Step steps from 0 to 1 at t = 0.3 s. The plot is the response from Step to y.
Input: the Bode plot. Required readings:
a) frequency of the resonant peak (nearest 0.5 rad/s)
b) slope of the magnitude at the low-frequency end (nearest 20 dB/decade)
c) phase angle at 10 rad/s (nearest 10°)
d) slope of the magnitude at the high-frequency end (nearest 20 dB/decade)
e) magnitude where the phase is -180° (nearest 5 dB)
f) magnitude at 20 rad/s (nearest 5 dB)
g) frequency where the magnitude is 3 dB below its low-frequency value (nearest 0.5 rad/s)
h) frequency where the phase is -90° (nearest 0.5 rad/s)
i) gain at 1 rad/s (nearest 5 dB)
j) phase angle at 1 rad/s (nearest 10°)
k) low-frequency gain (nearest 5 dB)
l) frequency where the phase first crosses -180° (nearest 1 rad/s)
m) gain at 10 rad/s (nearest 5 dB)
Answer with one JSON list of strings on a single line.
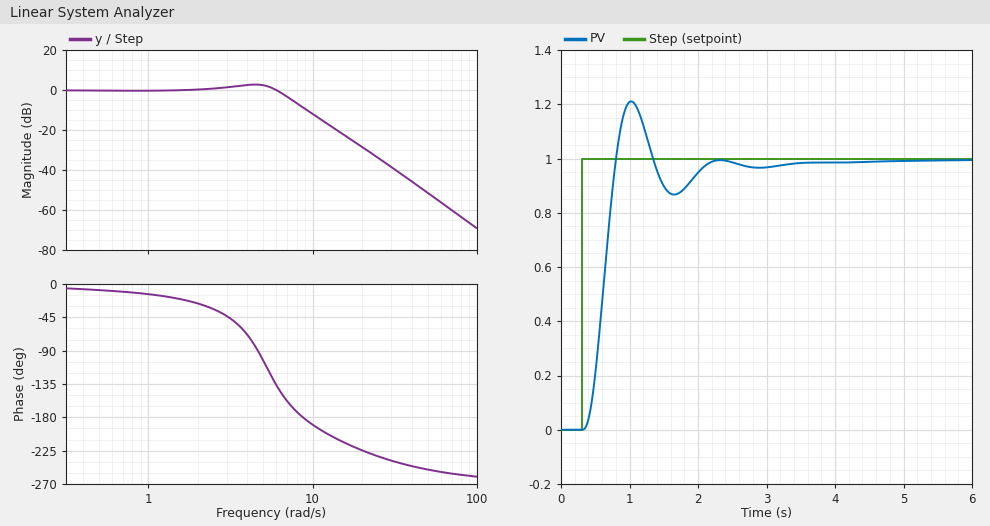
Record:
["4.5 rad/s", "0 dB/decade", "-190°", "-60 dB/decade", "-10 dB", "-30 dB", "7.0 rad/s", "4.5 rad/s", "0 dB", "-10°", "0 dB", "9 rad/s", "-10 dB"]
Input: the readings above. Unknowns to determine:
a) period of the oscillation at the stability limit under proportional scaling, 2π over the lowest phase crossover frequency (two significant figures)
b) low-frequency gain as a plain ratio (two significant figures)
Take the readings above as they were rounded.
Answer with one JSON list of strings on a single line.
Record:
["0.70 s", "1.0"]
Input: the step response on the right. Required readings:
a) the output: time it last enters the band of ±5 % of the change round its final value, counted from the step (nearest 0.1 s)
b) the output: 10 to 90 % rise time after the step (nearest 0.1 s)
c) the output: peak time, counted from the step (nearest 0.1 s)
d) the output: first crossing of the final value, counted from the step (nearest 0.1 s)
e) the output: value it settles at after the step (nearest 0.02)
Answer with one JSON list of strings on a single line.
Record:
["1.7 s", "0.3 s", "0.7 s", "0.5 s", "1.00"]
